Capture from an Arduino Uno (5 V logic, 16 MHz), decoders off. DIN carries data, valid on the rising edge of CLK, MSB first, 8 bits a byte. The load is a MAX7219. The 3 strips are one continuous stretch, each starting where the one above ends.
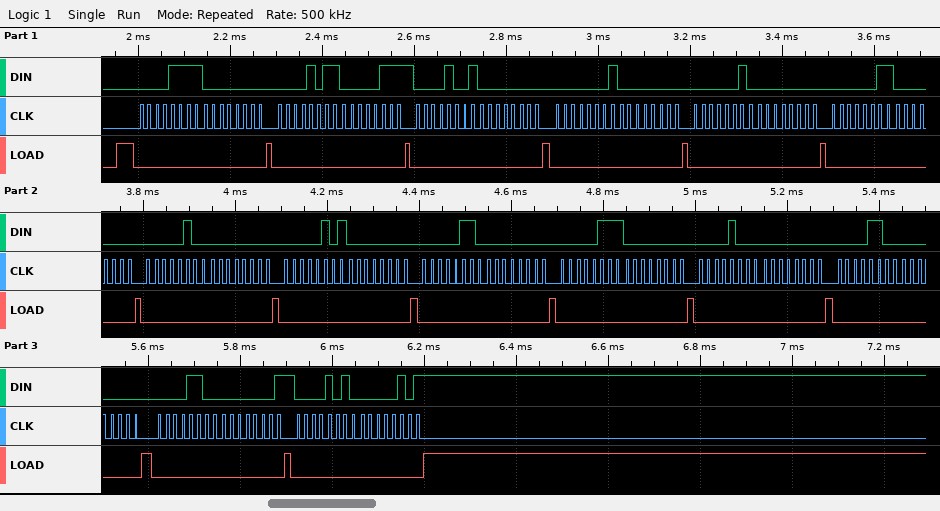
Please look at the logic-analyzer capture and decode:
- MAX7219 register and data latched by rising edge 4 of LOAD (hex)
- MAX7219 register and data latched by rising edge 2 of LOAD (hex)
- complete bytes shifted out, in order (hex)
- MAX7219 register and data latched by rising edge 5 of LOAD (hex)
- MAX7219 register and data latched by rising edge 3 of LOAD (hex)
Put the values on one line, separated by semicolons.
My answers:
register 0x9, data 0x00; register 0xF, data 0x00; 0x0F 0x00 0x0B 0x07 0x09 0x00 0x01 0x00 0x02 0x00 0x03 0x00 0x04 0x00 0x05 0x00 0x06 0x00 0x07 0x00 0x08 0x00 0x0C 0x00 0x0C 0x01 0x0A 0x05; register 0x1, data 0x00; register 0xB, data 0x07
